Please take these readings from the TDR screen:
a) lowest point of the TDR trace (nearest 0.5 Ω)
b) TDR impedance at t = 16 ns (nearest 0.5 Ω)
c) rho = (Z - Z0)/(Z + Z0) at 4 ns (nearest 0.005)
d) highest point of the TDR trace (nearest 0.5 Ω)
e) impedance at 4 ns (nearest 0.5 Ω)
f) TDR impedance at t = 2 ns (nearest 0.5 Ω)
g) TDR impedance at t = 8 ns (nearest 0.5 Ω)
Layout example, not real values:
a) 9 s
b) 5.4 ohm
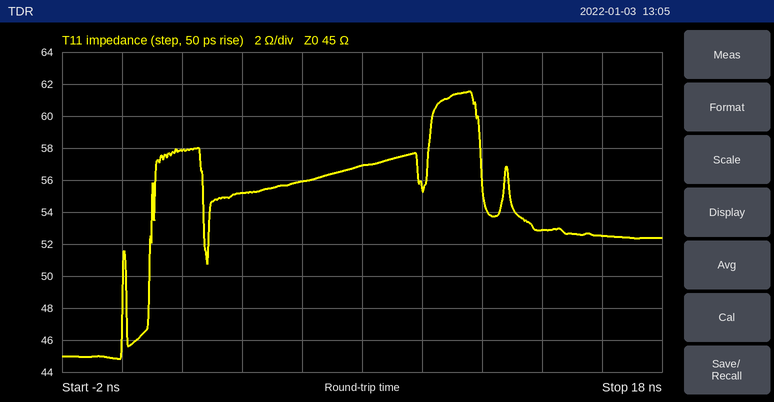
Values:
a) 45.0 Ω
b) 52.5 Ω
c) +0.100
d) 61.5 Ω
e) 55.0 Ω
f) 58.0 Ω
g) 57.0 Ω
